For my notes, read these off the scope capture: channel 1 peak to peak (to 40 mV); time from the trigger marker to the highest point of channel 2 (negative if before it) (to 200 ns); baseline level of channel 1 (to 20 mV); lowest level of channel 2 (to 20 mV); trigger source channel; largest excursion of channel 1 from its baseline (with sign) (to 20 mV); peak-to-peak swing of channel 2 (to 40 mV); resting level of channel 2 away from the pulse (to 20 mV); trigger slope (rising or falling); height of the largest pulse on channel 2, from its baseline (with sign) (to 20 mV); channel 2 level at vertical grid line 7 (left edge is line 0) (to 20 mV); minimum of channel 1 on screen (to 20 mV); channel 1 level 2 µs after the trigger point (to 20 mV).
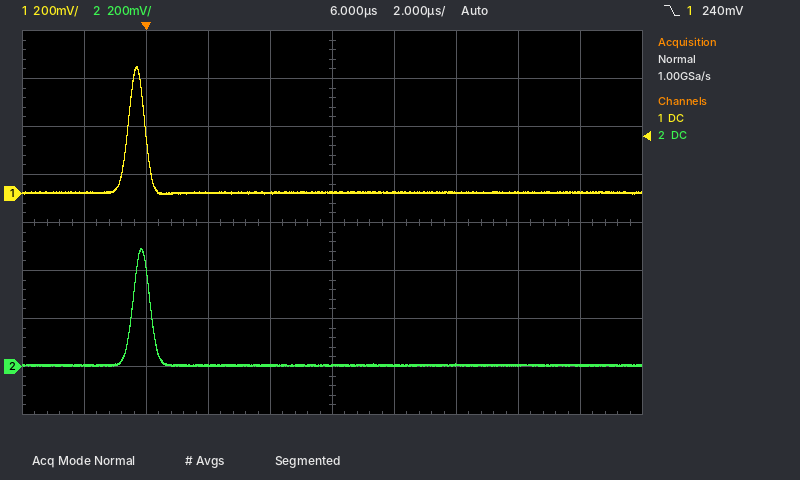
520 mV
-200 ns
0 mV
0 mV
channel 1
+520 mV
480 mV
0 mV
falling
+480 mV
0 mV
0 mV
0 mV
